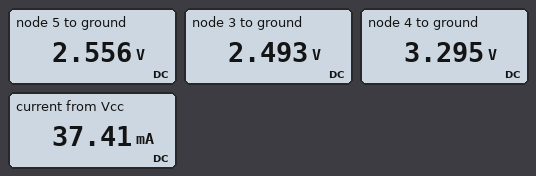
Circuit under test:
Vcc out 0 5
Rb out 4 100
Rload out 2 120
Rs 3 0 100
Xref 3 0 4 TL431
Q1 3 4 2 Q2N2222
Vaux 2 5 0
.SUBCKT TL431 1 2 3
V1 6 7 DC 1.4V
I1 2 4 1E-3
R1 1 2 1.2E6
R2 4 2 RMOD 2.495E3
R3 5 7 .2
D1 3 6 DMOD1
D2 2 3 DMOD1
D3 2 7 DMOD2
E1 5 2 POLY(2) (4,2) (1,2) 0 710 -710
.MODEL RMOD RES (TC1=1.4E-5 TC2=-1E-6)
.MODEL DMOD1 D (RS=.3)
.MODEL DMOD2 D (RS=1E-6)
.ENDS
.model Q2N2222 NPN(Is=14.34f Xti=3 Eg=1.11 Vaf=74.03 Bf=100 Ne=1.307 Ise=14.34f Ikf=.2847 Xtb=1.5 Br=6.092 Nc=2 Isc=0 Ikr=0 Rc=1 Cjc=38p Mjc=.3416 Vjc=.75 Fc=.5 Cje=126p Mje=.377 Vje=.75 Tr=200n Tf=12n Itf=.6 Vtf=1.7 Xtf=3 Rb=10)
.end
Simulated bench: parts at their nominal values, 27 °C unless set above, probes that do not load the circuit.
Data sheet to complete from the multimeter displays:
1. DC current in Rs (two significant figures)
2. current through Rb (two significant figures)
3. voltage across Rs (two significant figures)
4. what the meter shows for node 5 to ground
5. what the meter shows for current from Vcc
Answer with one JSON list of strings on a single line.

["25 mA", "17 mA", "2.5 V", "2.556 V", "37.41 mA"]
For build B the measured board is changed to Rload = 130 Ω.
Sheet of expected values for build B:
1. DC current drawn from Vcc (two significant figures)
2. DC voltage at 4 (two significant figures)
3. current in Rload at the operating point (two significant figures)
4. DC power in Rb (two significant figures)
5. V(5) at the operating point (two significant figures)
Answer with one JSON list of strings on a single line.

["36 mA", "3.3 V", "19 mA", "28 mW", "2.5 V"]
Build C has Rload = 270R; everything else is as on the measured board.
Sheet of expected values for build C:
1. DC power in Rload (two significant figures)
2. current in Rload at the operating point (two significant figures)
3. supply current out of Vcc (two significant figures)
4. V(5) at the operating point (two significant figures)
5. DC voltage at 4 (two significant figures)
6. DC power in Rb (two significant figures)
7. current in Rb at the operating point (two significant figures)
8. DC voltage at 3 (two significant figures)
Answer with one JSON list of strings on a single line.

["23 mW", "9.2 mA", "25 mA", "2.5 V", "3.4 V", "25 mW", "16 mA", "2.5 V"]
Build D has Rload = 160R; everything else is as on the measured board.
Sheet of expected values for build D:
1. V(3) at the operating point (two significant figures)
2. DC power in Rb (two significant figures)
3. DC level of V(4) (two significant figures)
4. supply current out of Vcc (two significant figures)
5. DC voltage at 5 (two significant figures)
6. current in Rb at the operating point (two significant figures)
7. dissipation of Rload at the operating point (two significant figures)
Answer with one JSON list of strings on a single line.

["2.5 V", "27 mW", "3.4 V", "32 mA", "2.5 V", "16 mA", "38 mW"]
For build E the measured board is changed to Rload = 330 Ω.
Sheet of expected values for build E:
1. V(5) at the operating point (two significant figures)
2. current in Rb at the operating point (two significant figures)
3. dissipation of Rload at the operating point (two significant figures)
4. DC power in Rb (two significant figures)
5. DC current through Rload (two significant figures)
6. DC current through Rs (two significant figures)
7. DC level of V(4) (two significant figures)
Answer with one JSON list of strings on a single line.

["2.4 V", "16 mA", "20 mW", "27 mW", "7.8 mA", "24 mA", "3.4 V"]
